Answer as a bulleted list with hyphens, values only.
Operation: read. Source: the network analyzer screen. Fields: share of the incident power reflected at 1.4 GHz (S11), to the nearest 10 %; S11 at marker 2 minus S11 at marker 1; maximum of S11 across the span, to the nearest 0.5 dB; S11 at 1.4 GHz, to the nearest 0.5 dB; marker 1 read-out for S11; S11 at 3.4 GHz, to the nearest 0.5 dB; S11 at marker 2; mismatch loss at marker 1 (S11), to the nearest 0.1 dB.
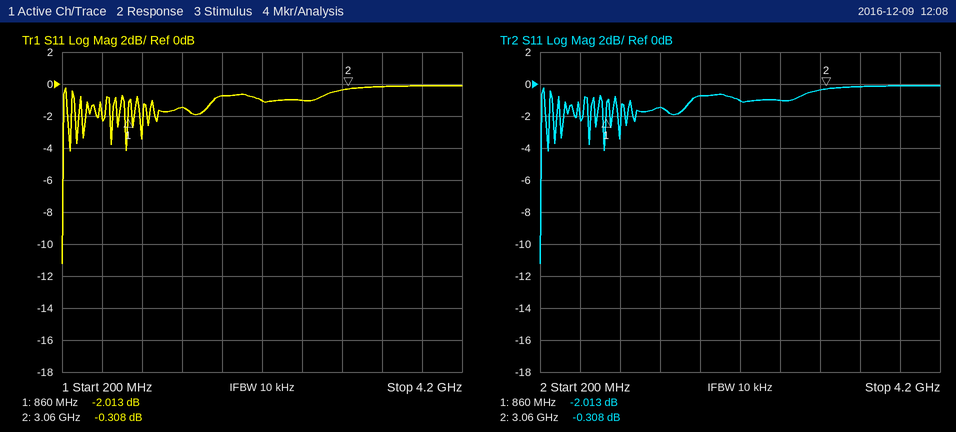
- 70 %
- 1.705 dB
- 0.0 dB
- -1.5 dB
- -2.013 dB
- 0.0 dB
- -0.308 dB
- 4.3 dB
